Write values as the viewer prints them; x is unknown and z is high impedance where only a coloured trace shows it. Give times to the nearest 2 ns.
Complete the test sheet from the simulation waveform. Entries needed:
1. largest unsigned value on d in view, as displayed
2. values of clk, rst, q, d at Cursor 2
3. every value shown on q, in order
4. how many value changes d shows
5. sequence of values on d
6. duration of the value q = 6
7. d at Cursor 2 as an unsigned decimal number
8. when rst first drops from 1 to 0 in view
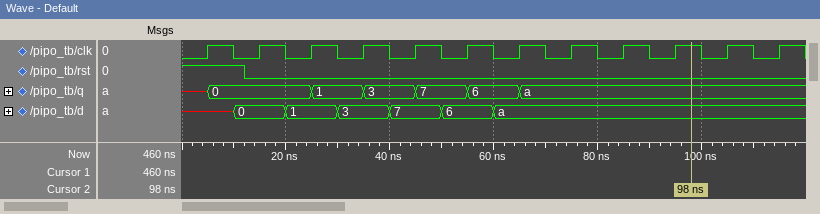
a
clk=1, rst=0, q=a, d=a
x, 0, 1, 3, 7, 6, a
6
x, 0, 1, 3, 7, 6, a
10 ns
10
12 ns
